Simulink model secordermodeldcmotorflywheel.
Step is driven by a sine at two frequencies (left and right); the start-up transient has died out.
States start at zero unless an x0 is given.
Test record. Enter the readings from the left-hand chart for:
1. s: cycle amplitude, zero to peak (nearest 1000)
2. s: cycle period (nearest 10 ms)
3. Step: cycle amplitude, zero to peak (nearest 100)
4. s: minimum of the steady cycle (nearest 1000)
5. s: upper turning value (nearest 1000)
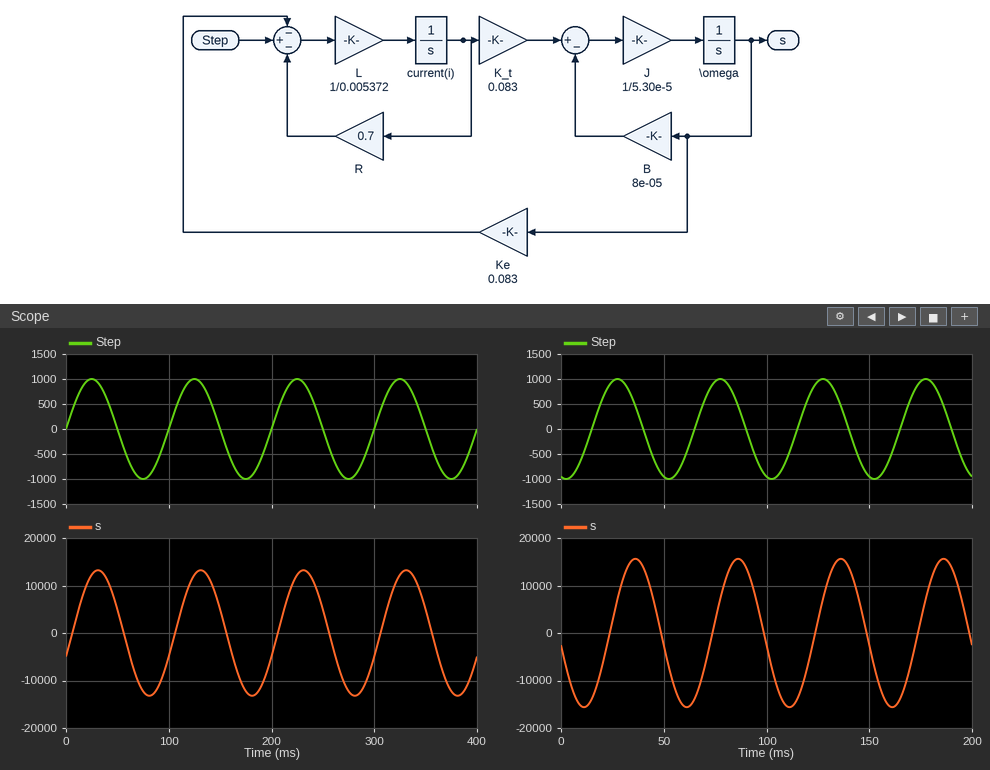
13000
100 ms
1000
-13000
13000
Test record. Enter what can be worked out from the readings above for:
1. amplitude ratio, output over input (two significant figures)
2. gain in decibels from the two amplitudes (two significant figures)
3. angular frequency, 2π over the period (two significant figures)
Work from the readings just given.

13
22 dB
0.063 rad/ms
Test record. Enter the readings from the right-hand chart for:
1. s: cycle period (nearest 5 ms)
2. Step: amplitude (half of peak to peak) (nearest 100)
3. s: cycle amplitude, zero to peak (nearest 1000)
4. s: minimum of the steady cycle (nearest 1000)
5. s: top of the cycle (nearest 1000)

50 ms
1000
16000
-16000
16000
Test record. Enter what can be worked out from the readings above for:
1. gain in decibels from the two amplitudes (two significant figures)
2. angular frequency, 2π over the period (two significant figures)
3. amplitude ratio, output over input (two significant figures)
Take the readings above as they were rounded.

24 dB
0.13 rad/ms
16
